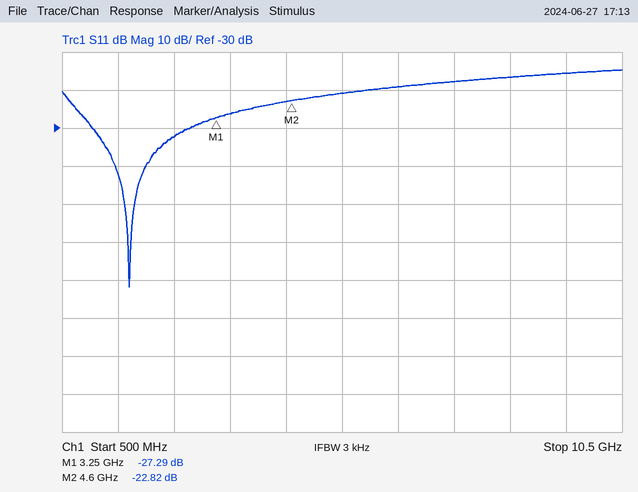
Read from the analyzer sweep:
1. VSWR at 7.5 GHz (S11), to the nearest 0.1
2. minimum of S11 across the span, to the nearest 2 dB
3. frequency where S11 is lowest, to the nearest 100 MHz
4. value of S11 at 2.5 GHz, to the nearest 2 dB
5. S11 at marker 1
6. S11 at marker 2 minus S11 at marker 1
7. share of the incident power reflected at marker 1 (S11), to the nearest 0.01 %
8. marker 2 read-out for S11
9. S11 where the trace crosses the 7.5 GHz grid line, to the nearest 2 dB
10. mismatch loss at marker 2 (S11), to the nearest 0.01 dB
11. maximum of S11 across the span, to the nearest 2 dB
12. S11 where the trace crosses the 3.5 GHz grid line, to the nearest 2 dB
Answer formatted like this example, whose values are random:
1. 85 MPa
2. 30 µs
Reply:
1. 1.3
2. -72 dB
3. 1.7 GHz
4. -32 dB
5. -27.29 dB
6. 4.47 dB
7. 0.19 %
8. -22.82 dB
9. -18 dB
10. 0.02 dB
11. -14 dB
12. -26 dB
